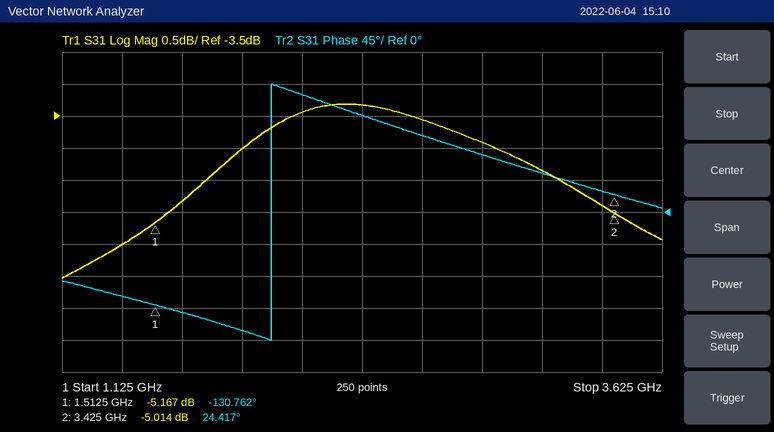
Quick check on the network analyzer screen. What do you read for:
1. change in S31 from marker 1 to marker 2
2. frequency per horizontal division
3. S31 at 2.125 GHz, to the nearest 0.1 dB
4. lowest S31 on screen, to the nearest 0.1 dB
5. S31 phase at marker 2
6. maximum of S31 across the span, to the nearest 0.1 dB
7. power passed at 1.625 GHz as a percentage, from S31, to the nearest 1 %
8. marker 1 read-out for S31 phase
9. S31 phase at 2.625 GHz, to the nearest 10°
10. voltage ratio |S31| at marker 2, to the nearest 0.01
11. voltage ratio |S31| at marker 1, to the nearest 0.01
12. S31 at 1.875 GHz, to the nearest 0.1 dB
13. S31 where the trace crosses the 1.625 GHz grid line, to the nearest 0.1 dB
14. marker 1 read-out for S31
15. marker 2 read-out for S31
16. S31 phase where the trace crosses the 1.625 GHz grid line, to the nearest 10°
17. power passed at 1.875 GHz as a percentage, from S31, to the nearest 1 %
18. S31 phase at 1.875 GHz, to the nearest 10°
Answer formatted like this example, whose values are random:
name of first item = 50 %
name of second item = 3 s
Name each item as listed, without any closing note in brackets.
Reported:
change in S31 from marker 1 to marker 2 = 0.153 dB
frequency per horizontal division = 250 MHz
S31 at 2.125 GHz, to the nearest 0.1 dB = -3.4 dB
lowest S31 on screen, to the nearest 0.1 dB = -6.0 dB
S31 phase at marker 2 = 24.417°
maximum of S31 across the span, to the nearest 0.1 dB = -3.3 dB
power passed at 1.625 GHz as a percentage, from S31, to the nearest 1 % = 33 %
marker 1 read-out for S31 phase = -130.762°
S31 phase at 2.625 GHz, to the nearest 10° = 110°
voltage ratio |S31| at marker 2, to the nearest 0.01 = 0.56
voltage ratio |S31| at marker 1, to the nearest 0.01 = 0.55
S31 at 1.875 GHz, to the nearest 0.1 dB = -4.0 dB
S31 where the trace crosses the 1.625 GHz grid line, to the nearest 0.1 dB = -4.8 dB
marker 1 read-out for S31 = -5.167 dB
marker 2 read-out for S31 = -5.014 dB
S31 phase where the trace crosses the 1.625 GHz grid line, to the nearest 10° = -140°
power passed at 1.875 GHz as a percentage, from S31, to the nearest 1 % = 40 %
S31 phase at 1.875 GHz, to the nearest 10° = -170°
